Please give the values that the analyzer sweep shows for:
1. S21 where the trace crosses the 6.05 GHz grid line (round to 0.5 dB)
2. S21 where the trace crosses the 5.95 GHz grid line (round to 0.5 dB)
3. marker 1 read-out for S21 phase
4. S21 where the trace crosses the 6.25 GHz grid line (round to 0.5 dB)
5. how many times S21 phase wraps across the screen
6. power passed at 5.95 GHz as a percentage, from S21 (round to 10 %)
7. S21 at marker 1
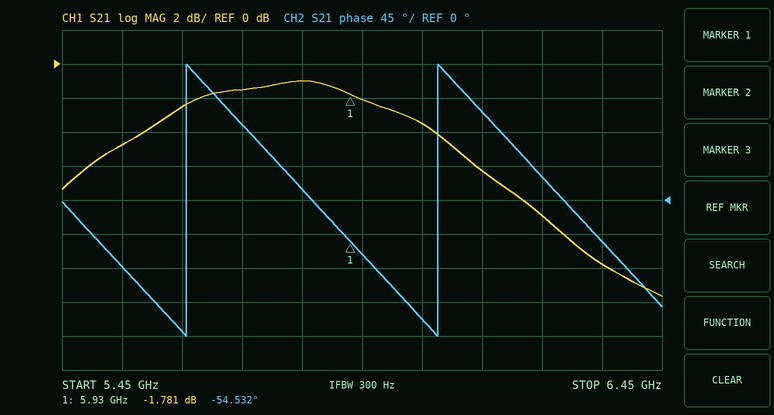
-3.5 dB
-2.0 dB
-54.532°
-9.0 dB
2
60 %
-1.781 dB
